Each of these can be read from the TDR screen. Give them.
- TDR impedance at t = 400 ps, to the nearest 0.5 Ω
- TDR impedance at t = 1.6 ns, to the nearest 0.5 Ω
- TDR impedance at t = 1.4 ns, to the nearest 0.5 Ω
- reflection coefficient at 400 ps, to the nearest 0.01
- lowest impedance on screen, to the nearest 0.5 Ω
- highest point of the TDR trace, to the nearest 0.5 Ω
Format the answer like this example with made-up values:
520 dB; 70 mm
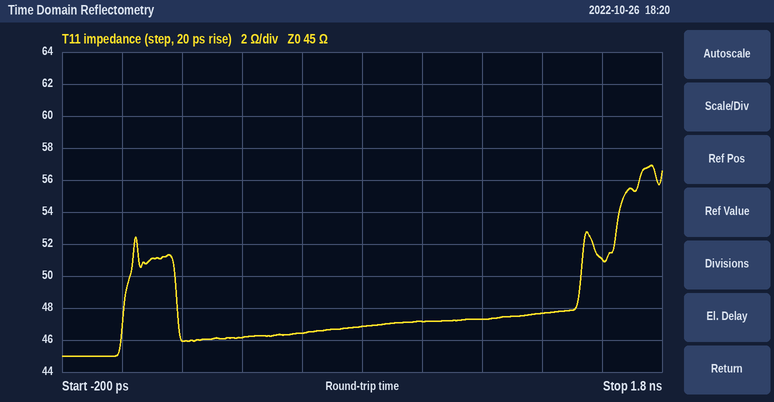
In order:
46.0 Ω; 51.0 Ω; 47.5 Ω; +0.01; 45.0 Ω; 57.0 Ω
